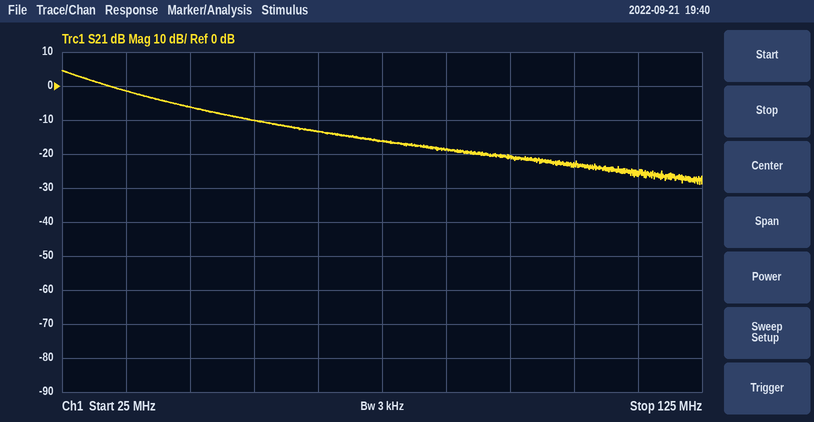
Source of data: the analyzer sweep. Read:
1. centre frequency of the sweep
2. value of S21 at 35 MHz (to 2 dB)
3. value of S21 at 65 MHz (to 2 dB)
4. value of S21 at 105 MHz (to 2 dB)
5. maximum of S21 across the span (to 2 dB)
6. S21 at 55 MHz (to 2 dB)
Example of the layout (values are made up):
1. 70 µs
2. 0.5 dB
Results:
1. 75 MHz
2. -2 dB
3. -14 dB
4. -24 dB
5. 4 dB
6. -10 dB
